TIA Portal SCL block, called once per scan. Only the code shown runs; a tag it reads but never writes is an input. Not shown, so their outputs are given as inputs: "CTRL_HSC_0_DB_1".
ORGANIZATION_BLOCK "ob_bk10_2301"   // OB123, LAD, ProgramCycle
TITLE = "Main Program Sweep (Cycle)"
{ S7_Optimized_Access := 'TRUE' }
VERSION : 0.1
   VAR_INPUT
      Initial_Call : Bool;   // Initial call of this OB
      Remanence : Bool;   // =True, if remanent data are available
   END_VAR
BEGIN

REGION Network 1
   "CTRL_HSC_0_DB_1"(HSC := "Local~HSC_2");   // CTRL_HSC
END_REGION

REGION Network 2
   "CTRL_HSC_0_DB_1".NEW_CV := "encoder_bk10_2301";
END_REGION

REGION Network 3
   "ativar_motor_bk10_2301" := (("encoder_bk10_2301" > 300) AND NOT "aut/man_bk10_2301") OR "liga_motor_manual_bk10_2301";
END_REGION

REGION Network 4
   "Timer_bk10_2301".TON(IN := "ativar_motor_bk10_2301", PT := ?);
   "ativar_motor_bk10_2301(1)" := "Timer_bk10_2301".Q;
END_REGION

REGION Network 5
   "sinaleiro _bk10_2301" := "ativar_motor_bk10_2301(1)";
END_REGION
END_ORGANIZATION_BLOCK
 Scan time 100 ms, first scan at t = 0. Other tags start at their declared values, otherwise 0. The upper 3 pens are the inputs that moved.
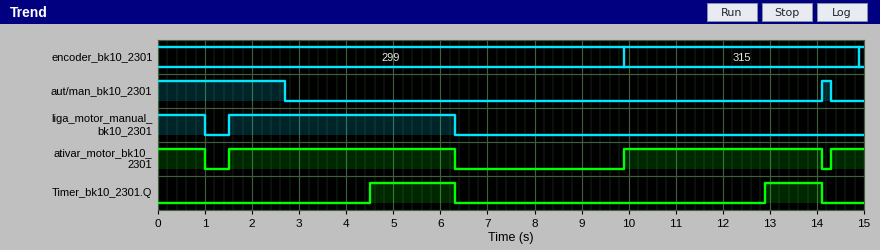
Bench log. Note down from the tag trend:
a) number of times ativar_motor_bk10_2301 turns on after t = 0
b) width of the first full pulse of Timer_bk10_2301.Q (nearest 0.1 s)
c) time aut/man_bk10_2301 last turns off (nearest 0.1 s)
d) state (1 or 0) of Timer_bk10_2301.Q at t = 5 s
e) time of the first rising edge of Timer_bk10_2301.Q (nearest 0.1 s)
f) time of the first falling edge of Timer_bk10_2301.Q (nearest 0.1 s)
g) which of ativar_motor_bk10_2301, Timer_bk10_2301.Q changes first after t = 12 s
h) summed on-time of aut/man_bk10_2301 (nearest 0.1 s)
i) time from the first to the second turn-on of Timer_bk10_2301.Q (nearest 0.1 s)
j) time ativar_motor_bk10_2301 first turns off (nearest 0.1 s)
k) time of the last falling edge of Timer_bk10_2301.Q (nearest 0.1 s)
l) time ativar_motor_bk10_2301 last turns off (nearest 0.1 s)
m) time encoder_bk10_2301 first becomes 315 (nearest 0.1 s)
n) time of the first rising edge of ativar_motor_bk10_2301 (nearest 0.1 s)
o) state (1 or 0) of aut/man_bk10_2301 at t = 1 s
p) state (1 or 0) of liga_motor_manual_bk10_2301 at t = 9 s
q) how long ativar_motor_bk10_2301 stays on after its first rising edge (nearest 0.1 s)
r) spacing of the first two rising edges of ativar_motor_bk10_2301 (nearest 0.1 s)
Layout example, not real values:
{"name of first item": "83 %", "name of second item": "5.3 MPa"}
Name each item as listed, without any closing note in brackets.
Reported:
{"number of times ativar_motor_bk10_2301 turns on after t = 0": "3", "width of the first full pulse of Timer_bk10_2301.Q": "1.8 s", "time aut/man_bk10_2301 last turns off": "14.3 s", "state (1 or 0) of Timer_bk10_2301.Q at t = 5 s": "1", "time of the first rising edge of Timer_bk10_2301.Q": "4.5 s", "time of the first falling edge of Timer_bk10_2301.Q": "6.3 s", "which of ativar_motor_bk10_2301, Timer_bk10_2301.Q changes first after t = 12 s": "Timer_bk10_2301.Q", "summed on-time of aut/man_bk10_2301": "2.9 s", "time from the first to the second turn-on of Timer_bk10_2301.Q": "8.4 s", "time ativar_motor_bk10_2301 first turns off": "1.0 s", "time of the last falling edge of Timer_bk10_2301.Q": "14.1 s", "time ativar_motor_bk10_2301 last turns off": "14.1 s", "time encoder_bk10_2301 first becomes 315": "9.9 s", "time of the first rising edge of ativar_motor_bk10_2301": "1.5 s", "state (1 or 0) of aut/man_bk10_2301 at t = 1 s": "1", "state (1 or 0) of liga_motor_manual_bk10_2301 at t = 9 s": "0", "how long ativar_motor_bk10_2301 stays on after its first rising edge": "4.8 s", "spacing of the first two rising edges of ativar_motor_bk10_2301": "8.4 s"}
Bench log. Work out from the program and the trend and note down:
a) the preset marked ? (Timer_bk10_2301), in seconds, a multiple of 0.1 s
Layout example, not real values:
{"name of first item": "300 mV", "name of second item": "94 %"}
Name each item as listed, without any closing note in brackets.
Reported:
{"the preset marked ? (Timer_bk10_2301), in seconds, a multiple of 0.1 s": "3.0 s"}
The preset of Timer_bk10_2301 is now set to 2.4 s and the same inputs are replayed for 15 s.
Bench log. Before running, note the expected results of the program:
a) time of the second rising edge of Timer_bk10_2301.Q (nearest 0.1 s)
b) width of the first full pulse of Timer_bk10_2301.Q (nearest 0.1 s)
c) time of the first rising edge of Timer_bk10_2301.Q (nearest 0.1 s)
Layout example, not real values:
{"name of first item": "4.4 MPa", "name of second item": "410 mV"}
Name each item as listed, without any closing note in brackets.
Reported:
{"time of the second rising edge of Timer_bk10_2301.Q": "12.3 s", "width of the first full pulse of Timer_bk10_2301.Q": "2.4 s", "time of the first rising edge of Timer_bk10_2301.Q": "3.9 s"}
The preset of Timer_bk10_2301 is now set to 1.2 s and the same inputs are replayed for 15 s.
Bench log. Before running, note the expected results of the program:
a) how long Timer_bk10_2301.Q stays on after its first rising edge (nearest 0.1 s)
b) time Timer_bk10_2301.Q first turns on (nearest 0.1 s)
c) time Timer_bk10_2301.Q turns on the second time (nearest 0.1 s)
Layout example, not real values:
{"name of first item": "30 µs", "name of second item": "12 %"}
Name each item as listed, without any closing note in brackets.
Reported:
{"how long Timer_bk10_2301.Q stays on after its first rising edge": "3.6 s", "time Timer_bk10_2301.Q first turns on": "2.7 s", "time Timer_bk10_2301.Q turns on the second time": "11.1 s"}
